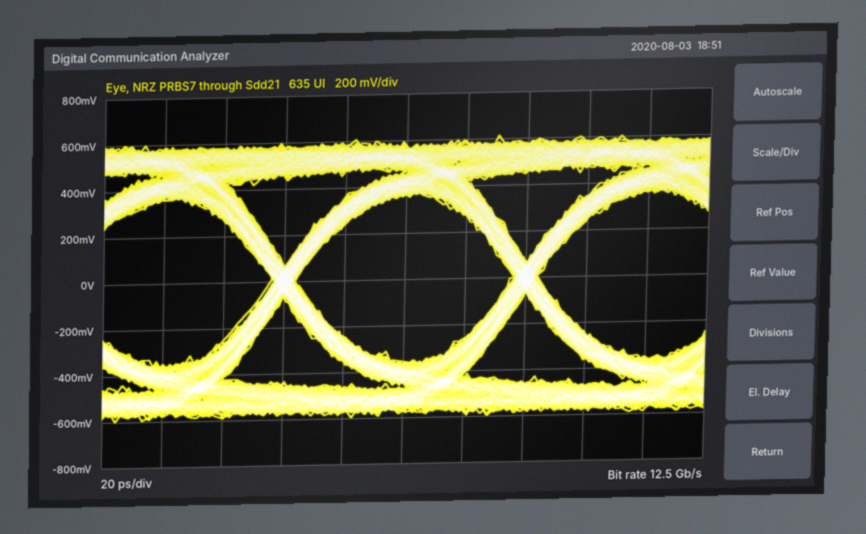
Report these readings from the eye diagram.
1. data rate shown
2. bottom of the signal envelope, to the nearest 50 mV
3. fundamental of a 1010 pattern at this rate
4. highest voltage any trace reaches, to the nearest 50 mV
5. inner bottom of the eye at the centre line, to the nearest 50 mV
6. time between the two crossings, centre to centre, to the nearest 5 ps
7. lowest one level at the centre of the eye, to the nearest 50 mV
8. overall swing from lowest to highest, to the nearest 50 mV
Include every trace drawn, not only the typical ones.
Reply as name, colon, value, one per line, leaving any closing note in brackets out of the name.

data rate shown: 12.5 Gb/s
bottom of the signal envelope, to the nearest 50 mV: -600 mV
fundamental of a 1010 pattern at this rate: 6.25 GHz
highest voltage any trace reaches, to the nearest 50 mV: 600 mV
inner bottom of the eye at the centre line, to the nearest 50 mV: -350 mV
time between the two crossings, centre to centre, to the nearest 5 ps: 80 ps
lowest one level at the centre of the eye, to the nearest 50 mV: 350 mV
overall swing from lowest to highest, to the nearest 50 mV: 1.20 V
